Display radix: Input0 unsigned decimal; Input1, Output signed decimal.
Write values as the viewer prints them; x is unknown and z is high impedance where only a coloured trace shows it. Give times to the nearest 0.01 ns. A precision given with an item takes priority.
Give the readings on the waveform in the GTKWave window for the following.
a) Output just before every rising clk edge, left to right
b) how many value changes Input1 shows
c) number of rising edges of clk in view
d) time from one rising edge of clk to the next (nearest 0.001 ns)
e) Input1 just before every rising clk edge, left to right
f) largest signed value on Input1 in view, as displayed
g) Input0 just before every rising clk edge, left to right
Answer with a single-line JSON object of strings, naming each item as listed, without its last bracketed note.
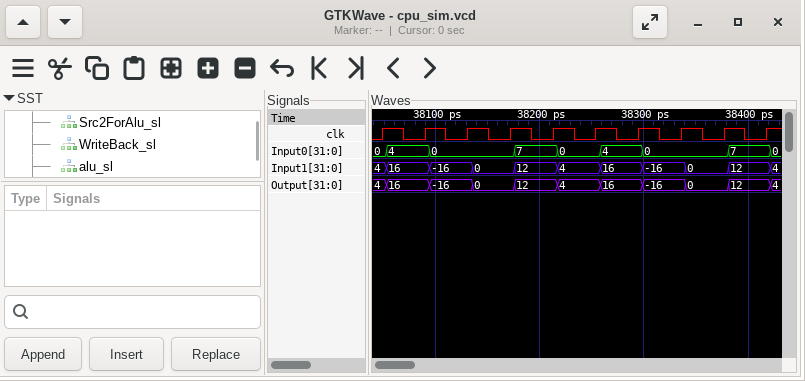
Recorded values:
{"Output just before every rising clk edge, left to right": "4, 16, -16, 0, 12, 4, 16, -16, 0, 12", "how many value changes Input1 shows": "10", "number of rising edges of clk in view": "10", "time from one rising edge of clk to the next": "0.041 ns", "Input1 just before every rising clk edge, left to right": "4, 16, -16, 0, 12, 4, 16, -16, 0, 12", "largest signed value on Input1 in view, as displayed": "16", "Input0 just before every rising clk edge, left to right": "0, 4, 0, 0, 7, 0, 4, 0, 0, 7"}
